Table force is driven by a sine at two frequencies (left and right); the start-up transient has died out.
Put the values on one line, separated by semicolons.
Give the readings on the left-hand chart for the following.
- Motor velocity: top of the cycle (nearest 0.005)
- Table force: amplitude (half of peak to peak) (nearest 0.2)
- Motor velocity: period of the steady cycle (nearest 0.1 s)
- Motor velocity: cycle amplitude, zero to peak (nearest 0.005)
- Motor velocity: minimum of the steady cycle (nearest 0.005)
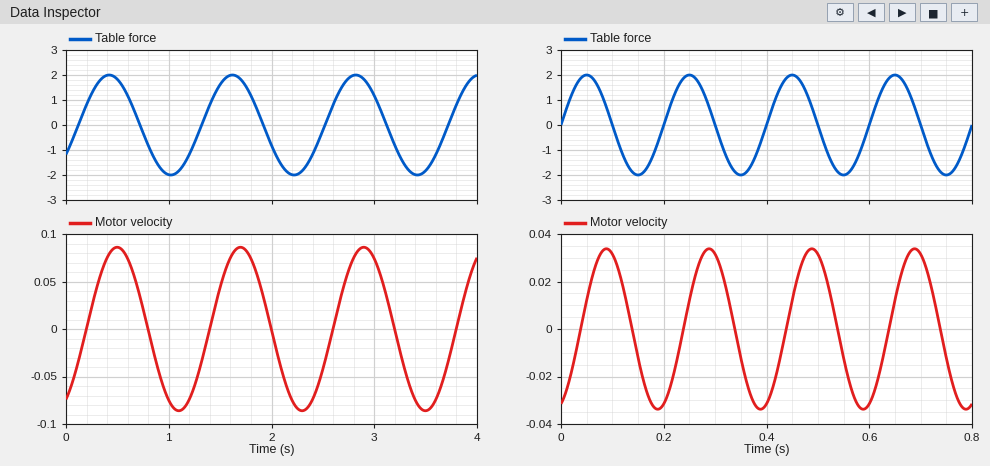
0.085; 2.0; 1.2 s; 0.085; -0.085
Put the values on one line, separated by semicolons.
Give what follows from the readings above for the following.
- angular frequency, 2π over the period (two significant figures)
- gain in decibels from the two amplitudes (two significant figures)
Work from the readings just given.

5.2 rad/s; -27 dB
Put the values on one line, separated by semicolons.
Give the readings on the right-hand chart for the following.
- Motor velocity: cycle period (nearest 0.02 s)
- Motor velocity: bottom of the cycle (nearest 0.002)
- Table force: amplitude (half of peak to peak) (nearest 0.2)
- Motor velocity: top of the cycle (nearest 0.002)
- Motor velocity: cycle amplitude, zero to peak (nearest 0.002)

0.20 s; -0.034; 2.0; 0.034; 0.034
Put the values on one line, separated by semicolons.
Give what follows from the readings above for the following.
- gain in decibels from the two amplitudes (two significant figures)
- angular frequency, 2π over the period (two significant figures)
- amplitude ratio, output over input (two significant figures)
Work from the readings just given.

-35 dB; 31 rad/s; 0.017
